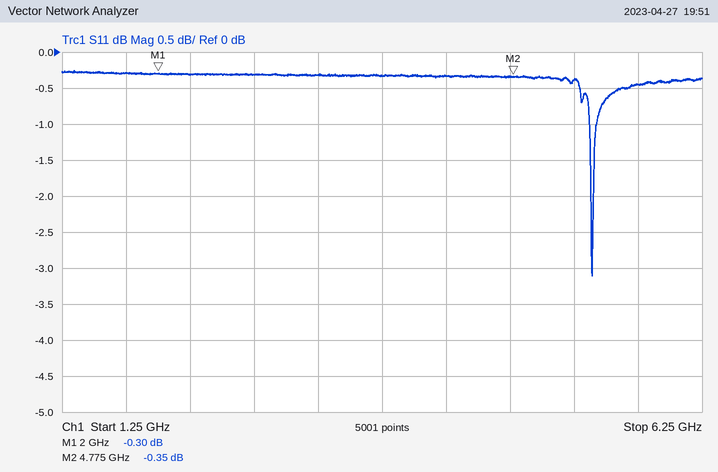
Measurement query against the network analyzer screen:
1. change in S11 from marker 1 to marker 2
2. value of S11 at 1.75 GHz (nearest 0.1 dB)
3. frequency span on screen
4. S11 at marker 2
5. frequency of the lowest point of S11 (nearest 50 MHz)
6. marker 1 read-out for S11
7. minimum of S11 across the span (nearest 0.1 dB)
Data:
-0.05 dB
-0.3 dB
5 GHz
-0.35 dB
5.40 GHz
-0.30 dB
-3.1 dB
